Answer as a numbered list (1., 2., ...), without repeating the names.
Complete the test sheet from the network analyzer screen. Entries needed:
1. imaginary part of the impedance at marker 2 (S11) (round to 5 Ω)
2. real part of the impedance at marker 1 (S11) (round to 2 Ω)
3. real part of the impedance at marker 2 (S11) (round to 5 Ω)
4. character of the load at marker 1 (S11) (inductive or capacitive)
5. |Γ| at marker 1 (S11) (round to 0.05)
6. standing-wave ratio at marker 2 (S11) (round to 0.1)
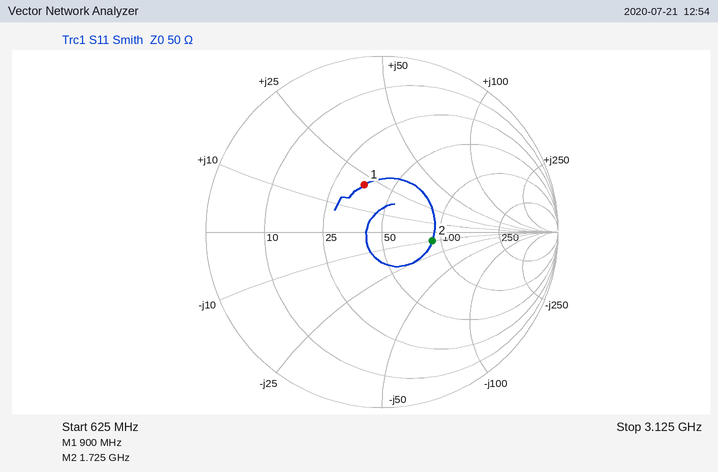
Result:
1. -10 Ω
2. 36 Ω
3. 90 Ω
4. inductive
5. 0.30
6. 1.8
